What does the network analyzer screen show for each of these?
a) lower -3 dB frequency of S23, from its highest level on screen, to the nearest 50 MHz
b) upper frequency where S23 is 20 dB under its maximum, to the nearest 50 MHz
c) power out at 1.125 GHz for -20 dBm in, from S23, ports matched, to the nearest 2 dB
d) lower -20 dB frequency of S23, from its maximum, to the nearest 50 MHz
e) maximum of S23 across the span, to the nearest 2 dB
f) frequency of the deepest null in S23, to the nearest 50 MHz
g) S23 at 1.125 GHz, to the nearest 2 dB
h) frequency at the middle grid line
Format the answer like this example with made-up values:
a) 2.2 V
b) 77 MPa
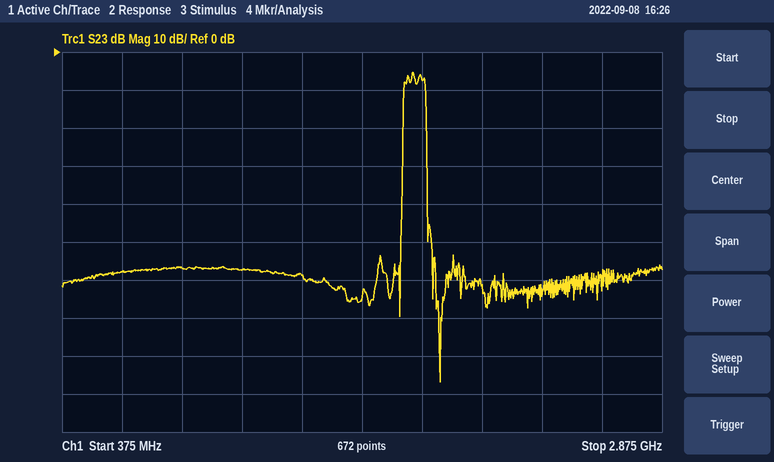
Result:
a) 1.80 GHz
b) 1.90 GHz
c) -78 dBm
d) 1.80 GHz
e) -6 dB
f) 1.95 GHz
g) -58 dB
h) 1.625 GHz
